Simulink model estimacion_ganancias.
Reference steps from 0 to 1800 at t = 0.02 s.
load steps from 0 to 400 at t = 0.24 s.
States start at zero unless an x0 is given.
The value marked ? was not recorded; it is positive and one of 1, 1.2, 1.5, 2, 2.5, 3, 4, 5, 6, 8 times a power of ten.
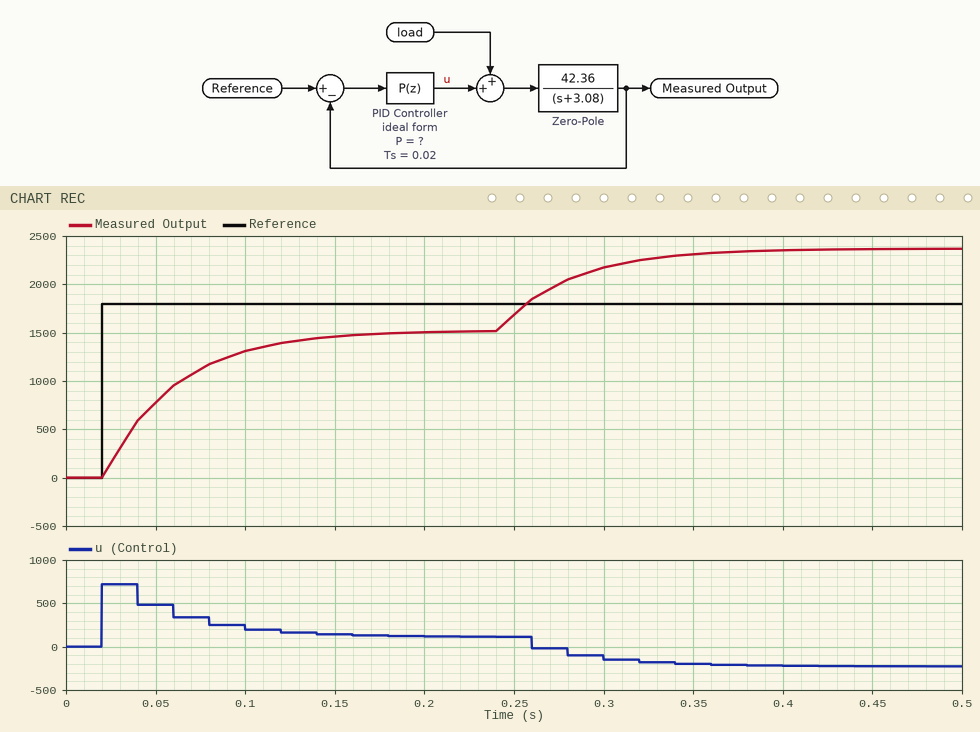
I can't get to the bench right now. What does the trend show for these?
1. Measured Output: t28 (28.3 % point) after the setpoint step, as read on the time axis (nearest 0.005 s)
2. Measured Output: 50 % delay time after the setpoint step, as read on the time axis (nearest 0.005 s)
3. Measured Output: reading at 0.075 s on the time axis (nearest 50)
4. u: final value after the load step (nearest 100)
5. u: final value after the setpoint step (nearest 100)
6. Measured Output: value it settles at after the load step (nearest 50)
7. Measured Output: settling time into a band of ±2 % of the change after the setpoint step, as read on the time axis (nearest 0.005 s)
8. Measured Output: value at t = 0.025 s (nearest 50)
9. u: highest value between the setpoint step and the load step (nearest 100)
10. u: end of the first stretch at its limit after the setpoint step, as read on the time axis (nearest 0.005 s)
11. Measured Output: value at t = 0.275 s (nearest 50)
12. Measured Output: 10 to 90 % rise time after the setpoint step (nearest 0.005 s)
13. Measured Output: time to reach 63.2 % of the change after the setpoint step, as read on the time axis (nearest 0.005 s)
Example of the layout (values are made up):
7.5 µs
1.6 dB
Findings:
0.035 s
0.050 s
1100
-200
100
2350
0.180 s
150
700
0.040 s
2000
0.090 s
0.060 s
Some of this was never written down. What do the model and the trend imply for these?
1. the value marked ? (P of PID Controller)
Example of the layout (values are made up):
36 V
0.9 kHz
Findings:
0.4
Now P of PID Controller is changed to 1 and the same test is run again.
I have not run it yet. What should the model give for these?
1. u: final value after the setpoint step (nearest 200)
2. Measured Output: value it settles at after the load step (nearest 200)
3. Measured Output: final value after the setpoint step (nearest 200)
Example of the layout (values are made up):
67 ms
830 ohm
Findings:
200
2000
1600
